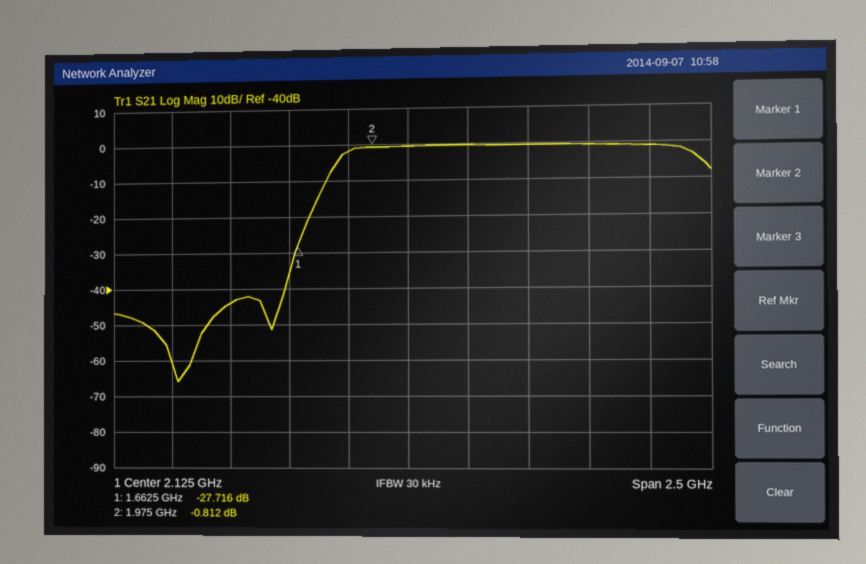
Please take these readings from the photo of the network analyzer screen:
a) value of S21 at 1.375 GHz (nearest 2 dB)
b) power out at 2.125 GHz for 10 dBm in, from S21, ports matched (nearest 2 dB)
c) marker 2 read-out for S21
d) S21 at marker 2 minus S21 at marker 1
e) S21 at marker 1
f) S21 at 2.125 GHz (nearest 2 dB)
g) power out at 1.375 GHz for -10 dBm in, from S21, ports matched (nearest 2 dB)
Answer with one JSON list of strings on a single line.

["-44 dB", "10 dBm", "-0.812 dB", "26.904 dB", "-27.716 dB", "0 dB", "-54 dBm"]
